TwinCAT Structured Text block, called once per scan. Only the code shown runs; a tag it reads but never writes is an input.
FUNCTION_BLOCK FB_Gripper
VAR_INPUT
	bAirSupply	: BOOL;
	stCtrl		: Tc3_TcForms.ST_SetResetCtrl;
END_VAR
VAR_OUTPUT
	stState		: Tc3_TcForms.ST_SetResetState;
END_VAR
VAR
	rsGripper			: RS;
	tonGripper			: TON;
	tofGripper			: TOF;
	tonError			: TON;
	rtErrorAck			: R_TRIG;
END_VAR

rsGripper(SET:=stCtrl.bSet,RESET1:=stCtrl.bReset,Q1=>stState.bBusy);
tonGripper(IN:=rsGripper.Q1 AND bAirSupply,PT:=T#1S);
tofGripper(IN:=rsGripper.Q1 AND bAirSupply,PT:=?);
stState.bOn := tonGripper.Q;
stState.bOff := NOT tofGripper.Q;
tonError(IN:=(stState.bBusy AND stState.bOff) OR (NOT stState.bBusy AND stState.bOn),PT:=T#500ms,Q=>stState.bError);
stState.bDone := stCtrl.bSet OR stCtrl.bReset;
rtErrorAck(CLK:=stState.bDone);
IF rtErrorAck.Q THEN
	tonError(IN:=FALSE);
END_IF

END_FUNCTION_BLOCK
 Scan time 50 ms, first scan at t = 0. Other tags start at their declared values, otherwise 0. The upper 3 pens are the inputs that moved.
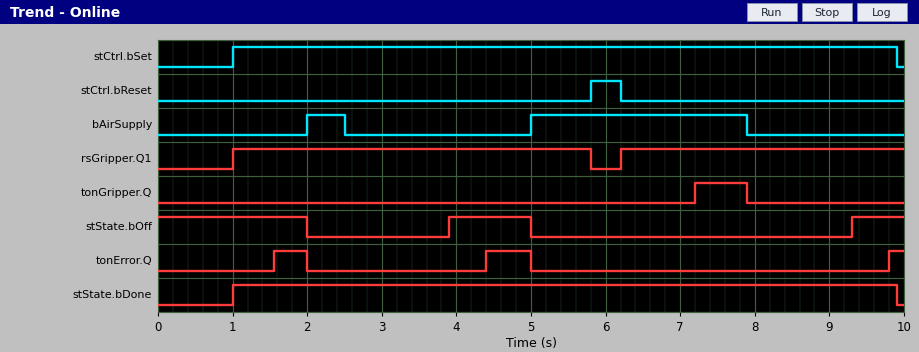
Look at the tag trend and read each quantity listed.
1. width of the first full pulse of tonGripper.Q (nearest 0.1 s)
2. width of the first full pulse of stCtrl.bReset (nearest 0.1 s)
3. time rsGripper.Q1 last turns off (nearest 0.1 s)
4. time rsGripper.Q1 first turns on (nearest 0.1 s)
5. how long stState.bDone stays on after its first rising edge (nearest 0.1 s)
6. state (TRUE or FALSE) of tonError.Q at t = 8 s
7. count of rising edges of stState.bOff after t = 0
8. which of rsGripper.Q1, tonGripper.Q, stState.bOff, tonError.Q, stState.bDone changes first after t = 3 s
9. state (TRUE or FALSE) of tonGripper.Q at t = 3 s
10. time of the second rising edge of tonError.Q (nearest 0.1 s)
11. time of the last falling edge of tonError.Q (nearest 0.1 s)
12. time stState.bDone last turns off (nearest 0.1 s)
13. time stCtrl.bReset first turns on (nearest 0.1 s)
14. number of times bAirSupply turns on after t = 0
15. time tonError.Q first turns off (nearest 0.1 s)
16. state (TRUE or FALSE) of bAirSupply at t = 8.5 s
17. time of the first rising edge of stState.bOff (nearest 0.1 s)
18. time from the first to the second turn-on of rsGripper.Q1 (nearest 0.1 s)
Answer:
0.7 s
0.4 s
5.8 s
1.0 s
8.9 s
FALSE
2
stState.bOff
FALSE
4.4 s
5.0 s
9.9 s
5.8 s
2
2.0 s
FALSE
3.9 s
5.2 s
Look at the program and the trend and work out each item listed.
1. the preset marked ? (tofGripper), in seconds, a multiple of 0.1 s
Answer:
1.4 s
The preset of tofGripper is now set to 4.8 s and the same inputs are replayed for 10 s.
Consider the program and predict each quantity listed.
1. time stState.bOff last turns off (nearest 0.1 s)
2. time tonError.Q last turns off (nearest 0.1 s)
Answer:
2.0 s
2.0 s
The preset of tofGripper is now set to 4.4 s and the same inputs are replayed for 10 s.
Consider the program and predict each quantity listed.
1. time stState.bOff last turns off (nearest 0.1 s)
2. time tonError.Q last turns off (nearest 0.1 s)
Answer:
2.0 s
2.0 s
